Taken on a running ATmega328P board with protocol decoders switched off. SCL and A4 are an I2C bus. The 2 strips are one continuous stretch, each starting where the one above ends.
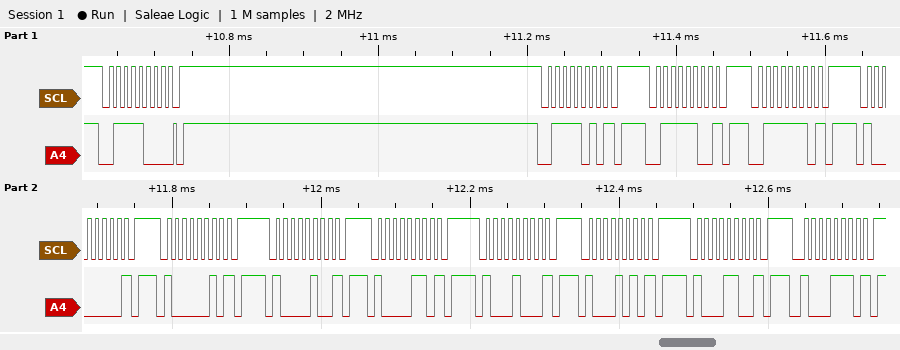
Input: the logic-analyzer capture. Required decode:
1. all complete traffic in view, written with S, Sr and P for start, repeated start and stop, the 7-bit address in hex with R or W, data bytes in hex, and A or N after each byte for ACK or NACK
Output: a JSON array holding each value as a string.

["S 3CW A P S 3DW N P S 3EW N P S 3FW N P S 40W N P S 41W N P S 42W N P S 43W N P S 44W N P S 45W N P S 46W N P S 47W N P"]
